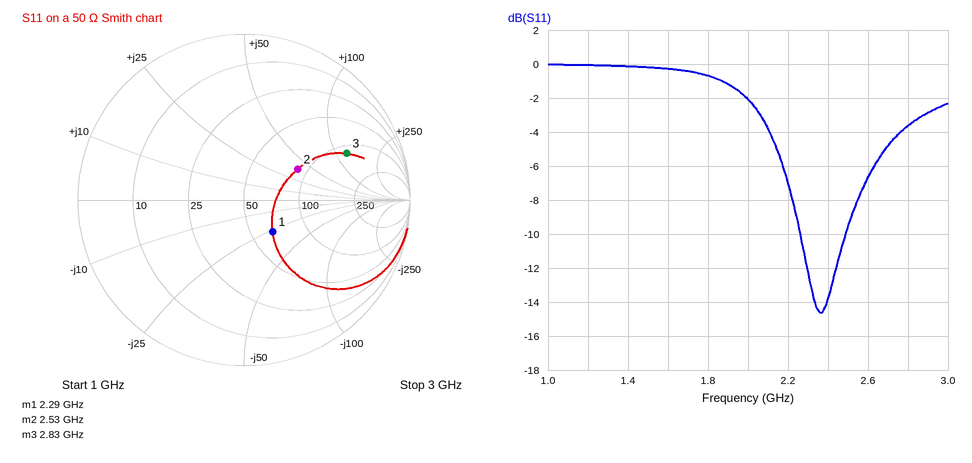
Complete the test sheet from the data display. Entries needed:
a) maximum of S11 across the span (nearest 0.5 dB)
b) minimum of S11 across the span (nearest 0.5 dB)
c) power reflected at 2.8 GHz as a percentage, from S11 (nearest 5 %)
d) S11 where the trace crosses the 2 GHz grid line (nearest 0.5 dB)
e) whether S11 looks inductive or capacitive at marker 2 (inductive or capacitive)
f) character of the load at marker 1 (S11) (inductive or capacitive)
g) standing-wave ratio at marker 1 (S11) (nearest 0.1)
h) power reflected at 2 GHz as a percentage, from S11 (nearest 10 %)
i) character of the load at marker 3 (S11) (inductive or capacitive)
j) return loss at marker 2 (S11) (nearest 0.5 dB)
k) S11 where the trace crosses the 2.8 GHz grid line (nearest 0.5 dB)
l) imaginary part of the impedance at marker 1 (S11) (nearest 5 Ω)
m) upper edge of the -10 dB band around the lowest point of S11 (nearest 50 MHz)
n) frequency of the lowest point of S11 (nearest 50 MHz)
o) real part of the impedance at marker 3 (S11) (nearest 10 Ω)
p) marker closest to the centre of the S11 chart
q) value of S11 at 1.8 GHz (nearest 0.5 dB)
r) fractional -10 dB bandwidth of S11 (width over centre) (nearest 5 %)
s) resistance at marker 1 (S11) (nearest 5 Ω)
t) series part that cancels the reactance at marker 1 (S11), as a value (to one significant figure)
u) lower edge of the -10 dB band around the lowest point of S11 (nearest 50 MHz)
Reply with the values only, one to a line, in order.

0.0 dB
-14.5 dB
45 %
-2.0 dB
inductive
capacitive
1.7
60 %
inductive
8.5 dB
-3.5 dB
-25 Ω
2.50 GHz
2.35 GHz
120 Ω
marker 1
-0.5 dB
10 %
65 Ω
2 nH
2.25 GHz
